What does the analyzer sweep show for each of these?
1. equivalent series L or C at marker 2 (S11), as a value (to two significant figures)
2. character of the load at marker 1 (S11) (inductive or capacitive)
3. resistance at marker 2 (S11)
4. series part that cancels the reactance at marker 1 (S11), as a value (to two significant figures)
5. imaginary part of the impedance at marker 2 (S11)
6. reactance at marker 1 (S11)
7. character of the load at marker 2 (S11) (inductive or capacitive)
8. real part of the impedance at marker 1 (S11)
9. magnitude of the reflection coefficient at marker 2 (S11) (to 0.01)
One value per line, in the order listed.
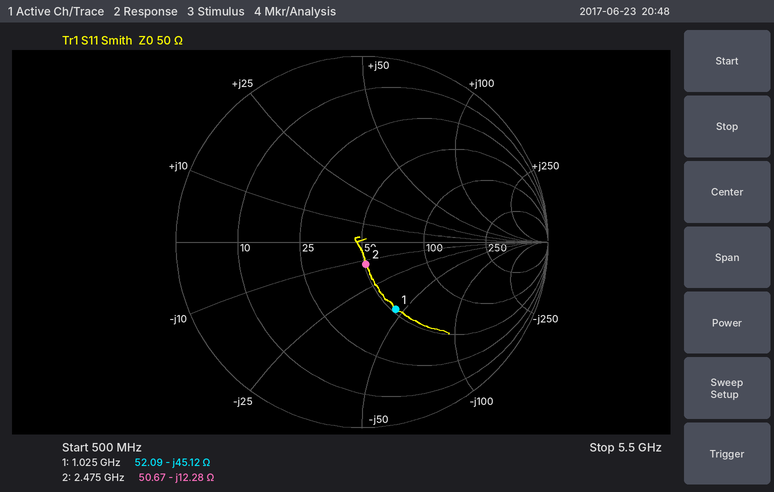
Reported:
5.2 pF
capacitive
50.67 Ω
7.0 nH
-12.28 Ω
-45.12 Ω
capacitive
52.09 Ω
0.12
